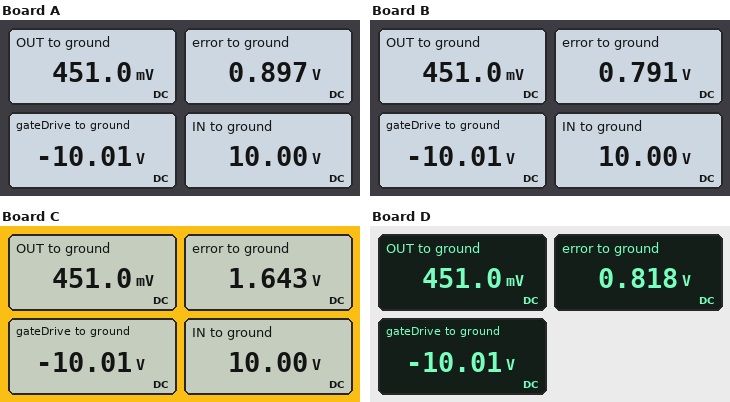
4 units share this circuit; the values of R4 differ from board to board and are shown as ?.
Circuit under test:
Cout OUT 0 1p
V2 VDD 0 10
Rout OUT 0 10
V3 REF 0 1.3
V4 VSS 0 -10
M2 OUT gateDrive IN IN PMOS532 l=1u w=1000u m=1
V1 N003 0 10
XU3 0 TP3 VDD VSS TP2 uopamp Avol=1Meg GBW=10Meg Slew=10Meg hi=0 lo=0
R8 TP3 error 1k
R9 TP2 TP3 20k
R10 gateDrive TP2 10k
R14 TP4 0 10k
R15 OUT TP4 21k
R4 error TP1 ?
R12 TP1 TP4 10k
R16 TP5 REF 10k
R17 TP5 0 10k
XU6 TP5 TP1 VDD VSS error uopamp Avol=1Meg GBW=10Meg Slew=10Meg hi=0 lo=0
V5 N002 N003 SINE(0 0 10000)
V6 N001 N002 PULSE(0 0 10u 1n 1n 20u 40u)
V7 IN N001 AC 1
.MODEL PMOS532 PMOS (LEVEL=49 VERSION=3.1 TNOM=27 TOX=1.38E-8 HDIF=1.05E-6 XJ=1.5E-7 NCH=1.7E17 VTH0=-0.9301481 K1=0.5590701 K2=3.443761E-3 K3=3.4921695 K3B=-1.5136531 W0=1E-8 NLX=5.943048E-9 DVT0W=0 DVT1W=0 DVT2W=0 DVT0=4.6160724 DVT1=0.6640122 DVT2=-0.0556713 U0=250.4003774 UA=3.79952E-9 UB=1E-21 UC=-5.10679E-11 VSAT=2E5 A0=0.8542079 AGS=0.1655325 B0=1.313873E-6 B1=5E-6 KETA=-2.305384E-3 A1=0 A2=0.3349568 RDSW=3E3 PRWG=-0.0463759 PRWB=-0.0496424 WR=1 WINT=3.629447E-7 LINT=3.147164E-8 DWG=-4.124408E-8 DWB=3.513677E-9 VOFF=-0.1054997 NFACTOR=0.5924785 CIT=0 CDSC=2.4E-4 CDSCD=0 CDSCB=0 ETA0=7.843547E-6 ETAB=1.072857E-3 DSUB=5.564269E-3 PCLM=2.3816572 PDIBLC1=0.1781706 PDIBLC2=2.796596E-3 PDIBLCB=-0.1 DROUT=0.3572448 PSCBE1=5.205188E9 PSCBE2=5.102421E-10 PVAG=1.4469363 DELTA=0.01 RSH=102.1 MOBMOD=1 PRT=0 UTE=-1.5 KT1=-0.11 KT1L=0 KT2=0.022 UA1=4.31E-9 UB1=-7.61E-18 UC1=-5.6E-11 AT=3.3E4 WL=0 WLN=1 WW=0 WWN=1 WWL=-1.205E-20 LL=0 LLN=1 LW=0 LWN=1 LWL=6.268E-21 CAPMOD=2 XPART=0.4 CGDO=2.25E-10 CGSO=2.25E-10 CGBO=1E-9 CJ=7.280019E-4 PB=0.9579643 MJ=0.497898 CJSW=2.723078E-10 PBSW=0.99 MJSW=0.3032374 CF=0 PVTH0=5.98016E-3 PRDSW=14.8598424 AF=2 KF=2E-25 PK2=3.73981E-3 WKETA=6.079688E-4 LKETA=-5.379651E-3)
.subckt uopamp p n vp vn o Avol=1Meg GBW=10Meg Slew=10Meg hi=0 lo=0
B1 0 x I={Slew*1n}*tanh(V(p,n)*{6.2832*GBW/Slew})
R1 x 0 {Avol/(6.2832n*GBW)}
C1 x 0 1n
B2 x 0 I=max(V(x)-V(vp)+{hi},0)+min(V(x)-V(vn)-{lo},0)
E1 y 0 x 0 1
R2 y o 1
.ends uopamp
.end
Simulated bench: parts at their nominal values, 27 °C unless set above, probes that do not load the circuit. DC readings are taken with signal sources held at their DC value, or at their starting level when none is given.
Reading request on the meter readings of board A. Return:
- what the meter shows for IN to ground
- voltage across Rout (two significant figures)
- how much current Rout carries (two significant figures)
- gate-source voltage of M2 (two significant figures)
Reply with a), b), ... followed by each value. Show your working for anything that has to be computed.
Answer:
a) 10.00 V
b) 451 mV = 450 mV
c) (451 mV) / 10 Ω = 45 mA
d) -10.01 V - 10 V = -20 V
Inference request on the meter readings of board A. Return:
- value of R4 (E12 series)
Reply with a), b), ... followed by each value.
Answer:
a) 8.2 kΩ
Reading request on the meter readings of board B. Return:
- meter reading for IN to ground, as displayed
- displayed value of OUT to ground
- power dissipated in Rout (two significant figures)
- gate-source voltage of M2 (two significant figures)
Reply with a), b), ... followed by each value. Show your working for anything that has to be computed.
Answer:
a) 10.00 V
b) 451.0 mV
c) (451 mV)^2 / 10 Ω = 20 mW
d) -10.01 V - 10 V = -20 V
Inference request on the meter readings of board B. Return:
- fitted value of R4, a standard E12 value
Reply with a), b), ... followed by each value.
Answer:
a) 4.7 kΩ
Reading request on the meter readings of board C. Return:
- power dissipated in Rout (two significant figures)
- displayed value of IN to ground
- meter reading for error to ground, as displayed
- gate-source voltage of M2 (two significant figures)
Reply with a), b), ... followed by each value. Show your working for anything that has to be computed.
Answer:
a) (451 mV)^2 / 10 Ω = 20 mW
b) 10.00 V
c) 1.643 V
d) -10.01 V - 10 V = -20 V
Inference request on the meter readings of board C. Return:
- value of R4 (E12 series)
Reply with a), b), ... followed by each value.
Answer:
a) 33 kΩ
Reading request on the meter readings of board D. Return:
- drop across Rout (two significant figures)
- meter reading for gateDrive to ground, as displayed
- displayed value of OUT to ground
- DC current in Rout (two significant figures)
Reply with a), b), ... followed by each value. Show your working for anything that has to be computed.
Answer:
a) 451 mV = 450 mV
b) -10.01 V
c) 451.0 mV
d) (451 mV) / 10 Ω = 45 mA
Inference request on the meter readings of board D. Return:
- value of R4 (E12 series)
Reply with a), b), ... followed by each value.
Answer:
a) 5.6 kΩ
